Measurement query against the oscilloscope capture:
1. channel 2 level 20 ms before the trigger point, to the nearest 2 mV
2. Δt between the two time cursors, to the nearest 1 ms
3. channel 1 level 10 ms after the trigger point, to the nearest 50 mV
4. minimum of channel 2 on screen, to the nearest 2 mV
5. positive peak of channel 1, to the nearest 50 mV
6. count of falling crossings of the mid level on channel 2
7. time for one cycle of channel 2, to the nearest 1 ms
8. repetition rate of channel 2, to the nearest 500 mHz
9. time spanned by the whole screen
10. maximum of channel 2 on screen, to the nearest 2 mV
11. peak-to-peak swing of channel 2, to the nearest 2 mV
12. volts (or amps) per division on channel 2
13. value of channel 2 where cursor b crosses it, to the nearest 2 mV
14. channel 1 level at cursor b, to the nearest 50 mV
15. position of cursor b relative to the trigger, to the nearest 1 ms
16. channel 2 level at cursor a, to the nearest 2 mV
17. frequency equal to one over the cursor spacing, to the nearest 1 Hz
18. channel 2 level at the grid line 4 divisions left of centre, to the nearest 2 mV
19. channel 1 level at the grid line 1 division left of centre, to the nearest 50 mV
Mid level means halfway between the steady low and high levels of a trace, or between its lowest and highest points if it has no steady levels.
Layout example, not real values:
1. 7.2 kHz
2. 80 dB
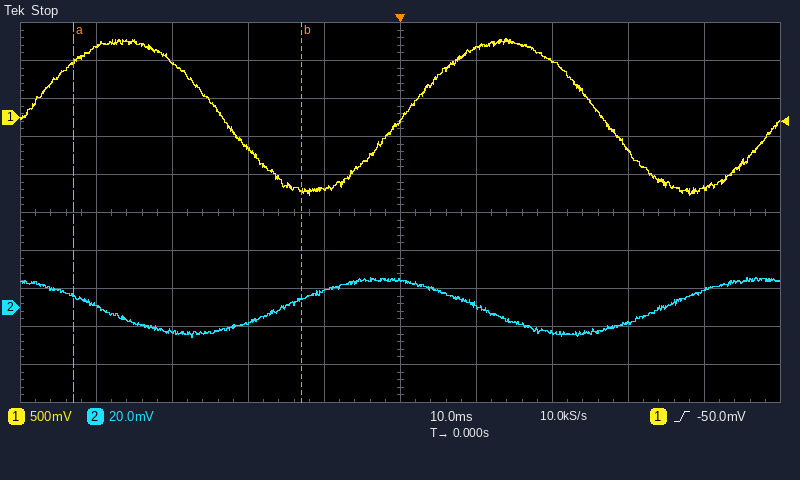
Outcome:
1. -8 mV
2. 30 ms
3. 900 mV
4. -16 mV
5. 1.05 V
6. 2
7. 50 ms
8. 20.0 Hz
9. 100 ms
10. 16 mV
11. 32 mV
12. 20 mV
13. 4 mV
14. -950 mV
15. -13 ms
16. 6 mV
17. 33 Hz
18. 2 mV
19. -950 mV
